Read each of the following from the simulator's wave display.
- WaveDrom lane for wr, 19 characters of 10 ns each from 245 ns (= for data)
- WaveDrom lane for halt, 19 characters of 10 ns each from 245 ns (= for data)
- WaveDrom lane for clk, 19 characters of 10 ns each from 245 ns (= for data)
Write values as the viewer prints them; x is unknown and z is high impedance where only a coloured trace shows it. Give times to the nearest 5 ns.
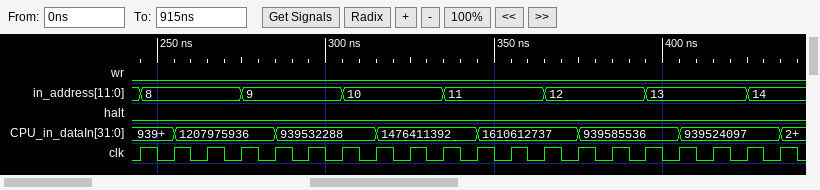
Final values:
{name: 'wr', wave: '0..................'}
{name: 'halt', wave: '0..................'}
{name: 'clk', wave: 'p..................'}
